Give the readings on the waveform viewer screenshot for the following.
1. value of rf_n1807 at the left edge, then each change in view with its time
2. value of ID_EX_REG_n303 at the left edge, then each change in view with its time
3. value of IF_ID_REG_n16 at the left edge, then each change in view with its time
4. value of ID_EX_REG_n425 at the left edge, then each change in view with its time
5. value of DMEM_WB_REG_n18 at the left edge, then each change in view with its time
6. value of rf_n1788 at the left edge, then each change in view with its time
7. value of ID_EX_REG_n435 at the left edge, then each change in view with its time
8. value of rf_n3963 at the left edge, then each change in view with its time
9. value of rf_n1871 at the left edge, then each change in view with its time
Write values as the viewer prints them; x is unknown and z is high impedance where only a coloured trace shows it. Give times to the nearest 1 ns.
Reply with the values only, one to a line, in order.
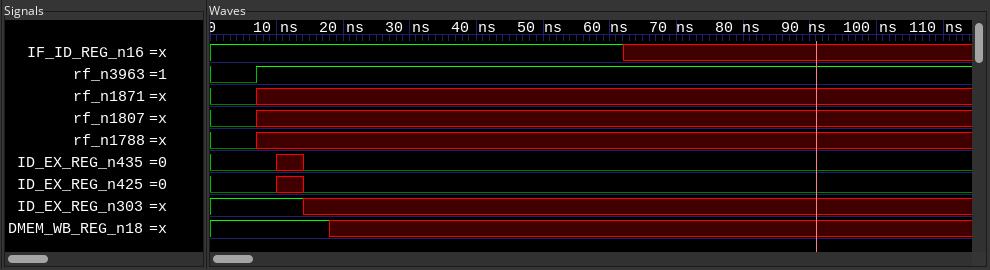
0, x at 7 ns
1, x at 14 ns
1, x at 62 ns
0, x at 10 ns, 0 at 14 ns
1, x at 18 ns
0, x at 7 ns
0, x at 10 ns, 0 at 14 ns
0, 1 at 7 ns
0, x at 7 ns
